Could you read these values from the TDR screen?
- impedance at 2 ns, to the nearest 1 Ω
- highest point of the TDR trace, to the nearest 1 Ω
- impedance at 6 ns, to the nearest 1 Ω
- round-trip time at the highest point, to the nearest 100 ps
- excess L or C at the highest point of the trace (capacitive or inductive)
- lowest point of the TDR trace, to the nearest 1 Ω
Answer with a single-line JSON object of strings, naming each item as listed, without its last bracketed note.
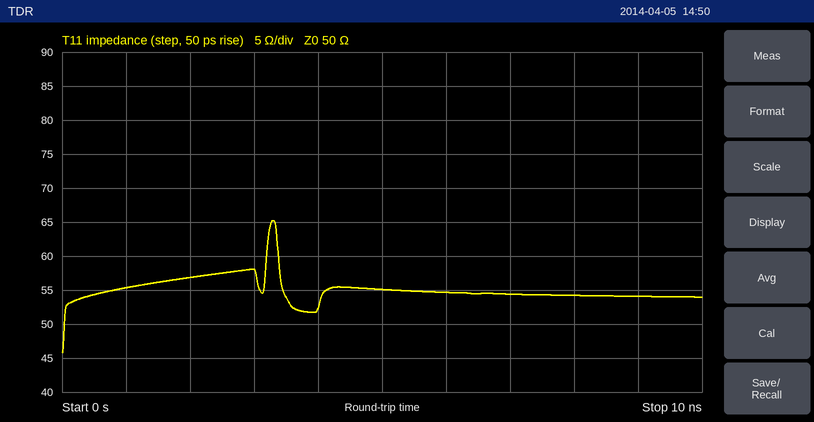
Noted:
{"impedance at 2 ns, to the nearest 1 Ω": "57 Ω", "highest point of the TDR trace, to the nearest 1 Ω": "65 Ω", "impedance at 6 ns, to the nearest 1 Ω": "55 Ω", "round-trip time at the highest point, to the nearest 100 ps": "3.3 ns", "excess L or C at the highest point of the trace": "inductive", "lowest point of the TDR trace, to the nearest 1 Ω": "46 Ω"}
